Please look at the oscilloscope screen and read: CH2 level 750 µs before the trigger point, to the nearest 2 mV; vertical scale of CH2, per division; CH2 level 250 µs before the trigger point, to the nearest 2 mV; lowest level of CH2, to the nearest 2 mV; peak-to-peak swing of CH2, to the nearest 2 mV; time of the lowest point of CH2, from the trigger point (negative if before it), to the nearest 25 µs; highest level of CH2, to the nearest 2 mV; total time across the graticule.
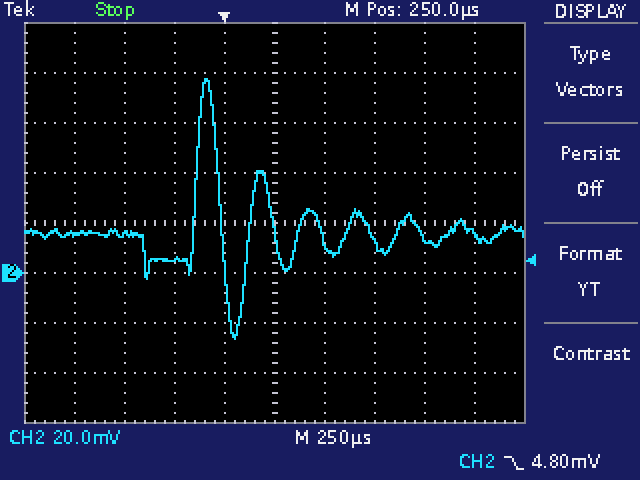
16 mV
20 mV
6 mV
-26 mV
104 mV
+50 µs
78 mV
2.5 ms
